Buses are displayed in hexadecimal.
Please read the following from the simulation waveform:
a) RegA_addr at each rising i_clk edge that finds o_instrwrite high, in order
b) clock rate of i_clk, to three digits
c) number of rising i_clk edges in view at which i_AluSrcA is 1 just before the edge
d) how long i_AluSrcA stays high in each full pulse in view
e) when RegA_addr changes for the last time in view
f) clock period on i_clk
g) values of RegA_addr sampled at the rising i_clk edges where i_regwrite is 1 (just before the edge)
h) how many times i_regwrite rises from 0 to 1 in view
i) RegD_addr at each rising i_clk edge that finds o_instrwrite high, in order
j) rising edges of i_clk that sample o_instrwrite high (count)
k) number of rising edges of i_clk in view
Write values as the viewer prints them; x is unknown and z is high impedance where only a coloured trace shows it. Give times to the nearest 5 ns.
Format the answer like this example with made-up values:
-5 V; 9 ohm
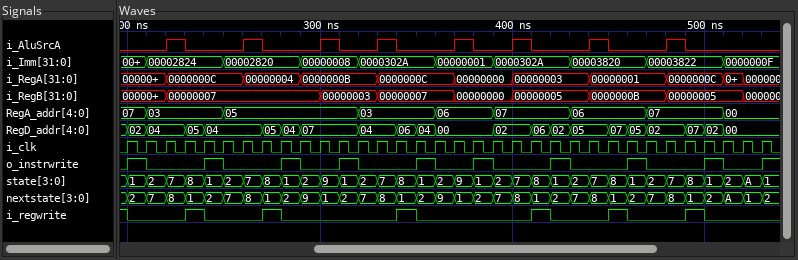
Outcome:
07, 03, 05, 05, 03, 06, 07, 06, 07; 100 MHz; 8; 10 ns, 10 ns, 10 ns, 10 ns, 10 ns, 10 ns, 10 ns, 10 ns; 510 ns; 10 ns; 07, 03, 05, 03, 07, 06, 07; 6; 02, 04, 04, 07, 04, 00, 02, 05, 02; 9; 34
